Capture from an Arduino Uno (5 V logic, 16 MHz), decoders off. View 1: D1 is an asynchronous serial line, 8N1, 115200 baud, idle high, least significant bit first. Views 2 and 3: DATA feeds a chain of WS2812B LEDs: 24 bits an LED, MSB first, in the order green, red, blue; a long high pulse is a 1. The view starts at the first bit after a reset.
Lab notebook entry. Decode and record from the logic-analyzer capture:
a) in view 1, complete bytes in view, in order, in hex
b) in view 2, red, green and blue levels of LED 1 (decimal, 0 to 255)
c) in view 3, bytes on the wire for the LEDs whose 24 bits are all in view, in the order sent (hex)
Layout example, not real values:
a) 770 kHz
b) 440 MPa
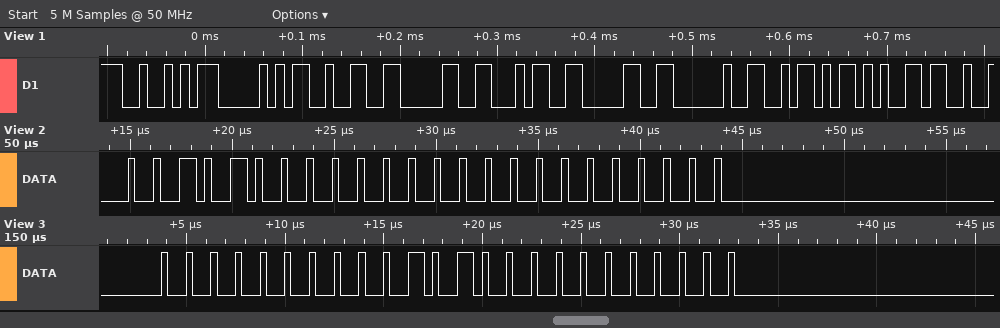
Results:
a) 52 50 32 30 34 30 20 5A 65
b) 0, 40, 0
c) 00 28 00
